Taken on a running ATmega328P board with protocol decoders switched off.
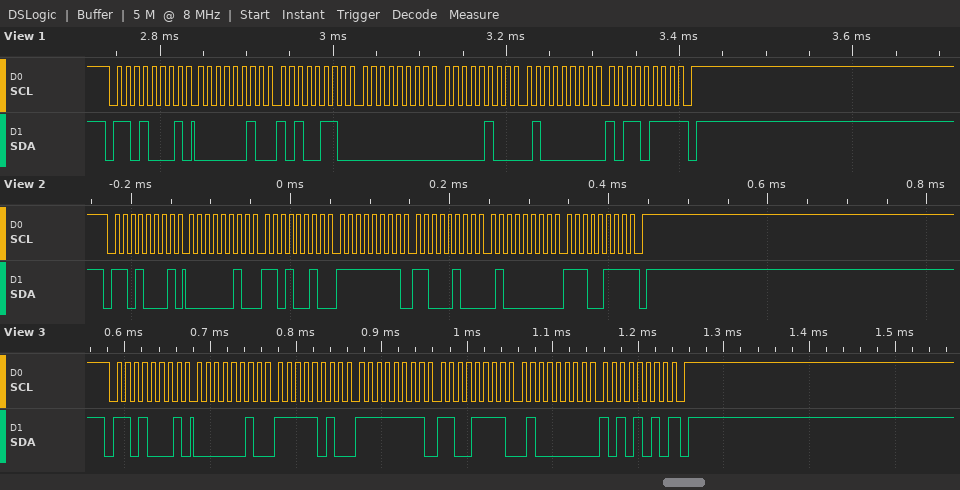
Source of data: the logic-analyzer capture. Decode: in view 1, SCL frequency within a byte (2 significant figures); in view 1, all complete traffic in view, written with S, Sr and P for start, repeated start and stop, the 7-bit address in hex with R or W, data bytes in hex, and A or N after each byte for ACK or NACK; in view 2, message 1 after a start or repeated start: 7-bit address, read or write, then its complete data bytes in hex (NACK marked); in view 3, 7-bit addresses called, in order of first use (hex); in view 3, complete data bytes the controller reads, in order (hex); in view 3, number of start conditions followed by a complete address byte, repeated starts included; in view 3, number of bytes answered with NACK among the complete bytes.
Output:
100 kHz
S 68R A 02 A A6 A 00 A 04 A 40 A B7 N P
0x68 read: 02 D2 FF C4 40 E7 NACK
0x68
02 FA FF CF 40 AA
1
1
